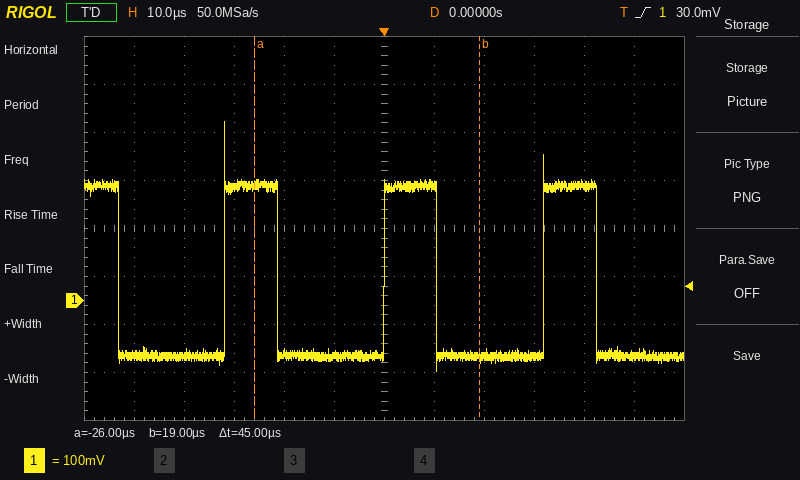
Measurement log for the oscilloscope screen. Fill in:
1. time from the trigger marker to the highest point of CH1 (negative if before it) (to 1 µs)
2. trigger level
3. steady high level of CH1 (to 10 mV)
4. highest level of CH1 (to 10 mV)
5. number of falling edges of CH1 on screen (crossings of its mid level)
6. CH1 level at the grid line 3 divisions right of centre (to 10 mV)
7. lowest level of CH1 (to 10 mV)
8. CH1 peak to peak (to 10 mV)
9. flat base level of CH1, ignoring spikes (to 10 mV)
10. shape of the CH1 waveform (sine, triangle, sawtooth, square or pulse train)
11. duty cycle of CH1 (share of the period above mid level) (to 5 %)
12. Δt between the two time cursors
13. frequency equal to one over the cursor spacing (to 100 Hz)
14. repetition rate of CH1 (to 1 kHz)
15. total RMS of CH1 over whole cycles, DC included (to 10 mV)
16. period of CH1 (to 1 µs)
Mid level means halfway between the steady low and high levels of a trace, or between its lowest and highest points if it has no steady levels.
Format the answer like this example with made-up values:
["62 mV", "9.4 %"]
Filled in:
["-32 µs", "30.0 mV", "240 mV", "370 mV", "4", "-120 mV", "-150 mV", "520 mV", "-120 mV", "pulse train", "35 %", "45 µs", "22.2 kHz", "31 kHz", "170 mV", "32 µs"]
